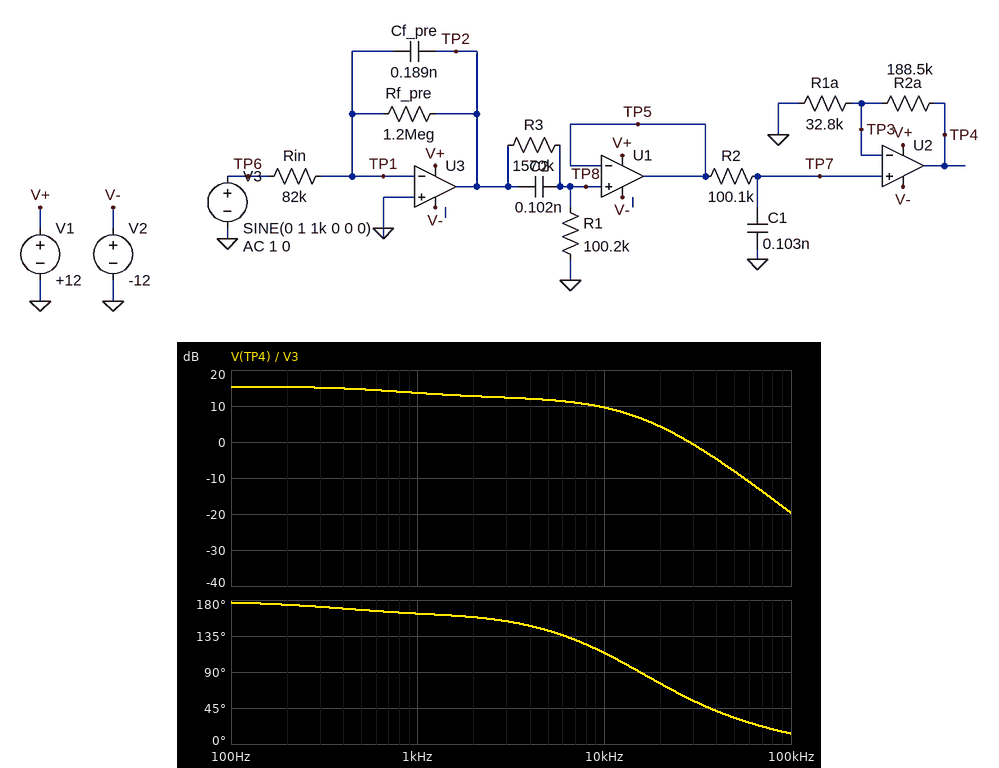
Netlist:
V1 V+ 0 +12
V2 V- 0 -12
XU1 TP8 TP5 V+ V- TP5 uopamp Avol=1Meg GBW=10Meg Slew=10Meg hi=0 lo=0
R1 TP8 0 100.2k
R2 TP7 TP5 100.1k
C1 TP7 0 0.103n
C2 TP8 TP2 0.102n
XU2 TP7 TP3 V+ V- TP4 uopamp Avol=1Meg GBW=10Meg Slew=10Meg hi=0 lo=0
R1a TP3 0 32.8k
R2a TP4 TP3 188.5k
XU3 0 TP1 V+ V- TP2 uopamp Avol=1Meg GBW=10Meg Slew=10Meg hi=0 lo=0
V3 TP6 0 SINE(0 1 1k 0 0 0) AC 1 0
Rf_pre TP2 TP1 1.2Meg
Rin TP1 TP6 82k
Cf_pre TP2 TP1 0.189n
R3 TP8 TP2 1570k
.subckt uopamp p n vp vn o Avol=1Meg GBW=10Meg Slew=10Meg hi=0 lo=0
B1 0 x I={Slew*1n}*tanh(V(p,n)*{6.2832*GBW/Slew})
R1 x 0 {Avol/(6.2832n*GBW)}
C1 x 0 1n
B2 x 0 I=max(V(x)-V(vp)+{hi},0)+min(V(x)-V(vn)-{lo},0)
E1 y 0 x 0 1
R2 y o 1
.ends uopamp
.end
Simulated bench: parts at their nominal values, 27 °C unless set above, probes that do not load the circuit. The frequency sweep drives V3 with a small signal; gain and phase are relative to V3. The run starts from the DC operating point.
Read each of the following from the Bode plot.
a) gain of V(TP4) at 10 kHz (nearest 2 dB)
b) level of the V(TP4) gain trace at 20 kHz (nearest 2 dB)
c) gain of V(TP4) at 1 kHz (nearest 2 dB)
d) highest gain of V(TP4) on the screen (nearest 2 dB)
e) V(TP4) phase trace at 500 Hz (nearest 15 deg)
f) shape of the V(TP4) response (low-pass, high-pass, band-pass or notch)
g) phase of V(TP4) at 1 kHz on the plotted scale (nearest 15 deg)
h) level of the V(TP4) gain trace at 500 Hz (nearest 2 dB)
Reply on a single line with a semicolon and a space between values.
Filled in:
10 dB; 4 dB; 14 dB; 16 dB; 165 deg; low-pass; 165 deg; 14 dB
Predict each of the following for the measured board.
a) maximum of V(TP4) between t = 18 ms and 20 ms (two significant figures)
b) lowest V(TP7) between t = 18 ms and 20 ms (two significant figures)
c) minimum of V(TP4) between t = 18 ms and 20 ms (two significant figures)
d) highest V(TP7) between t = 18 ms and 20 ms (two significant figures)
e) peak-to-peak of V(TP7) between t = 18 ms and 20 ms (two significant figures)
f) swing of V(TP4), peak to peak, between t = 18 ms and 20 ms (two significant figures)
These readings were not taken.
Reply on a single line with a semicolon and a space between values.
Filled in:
4.8 V; -710 mV; -4.8 V; 710 mV; 1.4 V; 9.6 V
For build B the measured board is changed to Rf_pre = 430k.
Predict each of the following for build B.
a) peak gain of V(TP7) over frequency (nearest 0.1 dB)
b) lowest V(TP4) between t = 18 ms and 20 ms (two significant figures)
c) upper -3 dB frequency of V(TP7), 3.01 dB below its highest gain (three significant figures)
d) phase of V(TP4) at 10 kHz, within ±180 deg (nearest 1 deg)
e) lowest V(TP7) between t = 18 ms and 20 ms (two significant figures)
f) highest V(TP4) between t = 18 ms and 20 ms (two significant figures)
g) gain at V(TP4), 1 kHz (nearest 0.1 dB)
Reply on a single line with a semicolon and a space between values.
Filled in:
-5.4 dB; -2.7 V; 12.5 kHz; 121 deg; -400 mV; 2.7 V; 8.5 dB
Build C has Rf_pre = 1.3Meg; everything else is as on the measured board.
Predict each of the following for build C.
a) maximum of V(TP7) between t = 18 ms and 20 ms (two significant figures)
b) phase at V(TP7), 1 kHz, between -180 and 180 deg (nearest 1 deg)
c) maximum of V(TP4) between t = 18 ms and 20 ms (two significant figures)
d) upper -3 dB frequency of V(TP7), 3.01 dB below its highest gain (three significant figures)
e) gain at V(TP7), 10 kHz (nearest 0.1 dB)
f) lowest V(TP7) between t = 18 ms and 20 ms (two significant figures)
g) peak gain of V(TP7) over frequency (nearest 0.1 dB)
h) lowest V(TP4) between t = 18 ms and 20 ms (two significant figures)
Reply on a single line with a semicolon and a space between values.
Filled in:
730 mV; 161 deg; 4.9 V; 1.55 kHz; -7.0 dB; -730 mV; -0.4 dB; -4.9 V
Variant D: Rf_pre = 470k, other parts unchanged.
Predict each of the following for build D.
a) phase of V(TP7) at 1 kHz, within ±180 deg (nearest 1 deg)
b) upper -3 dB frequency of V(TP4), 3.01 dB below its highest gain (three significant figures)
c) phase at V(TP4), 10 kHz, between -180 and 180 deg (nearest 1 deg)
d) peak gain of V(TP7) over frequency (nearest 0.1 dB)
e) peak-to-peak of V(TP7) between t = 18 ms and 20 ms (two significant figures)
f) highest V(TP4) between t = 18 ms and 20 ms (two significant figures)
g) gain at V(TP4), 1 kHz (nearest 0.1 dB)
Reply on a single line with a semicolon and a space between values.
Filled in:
-171 deg; 12.2 kHz; 120 deg; -5.2 dB; 850 mV; 2.9 V; 9.1 dB
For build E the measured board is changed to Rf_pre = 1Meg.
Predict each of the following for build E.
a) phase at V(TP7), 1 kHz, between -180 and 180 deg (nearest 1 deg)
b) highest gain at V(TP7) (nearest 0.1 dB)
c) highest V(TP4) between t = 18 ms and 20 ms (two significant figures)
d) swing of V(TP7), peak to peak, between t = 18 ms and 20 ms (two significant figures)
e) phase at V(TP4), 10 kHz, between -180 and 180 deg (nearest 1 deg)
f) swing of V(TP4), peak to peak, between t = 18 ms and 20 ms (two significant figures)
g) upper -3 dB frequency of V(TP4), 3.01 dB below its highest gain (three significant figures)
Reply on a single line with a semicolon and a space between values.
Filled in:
168 deg; -2.7 dB; 4.5 V; 1.3 V; 115 deg; 9.0 V; 7.15 kHz
